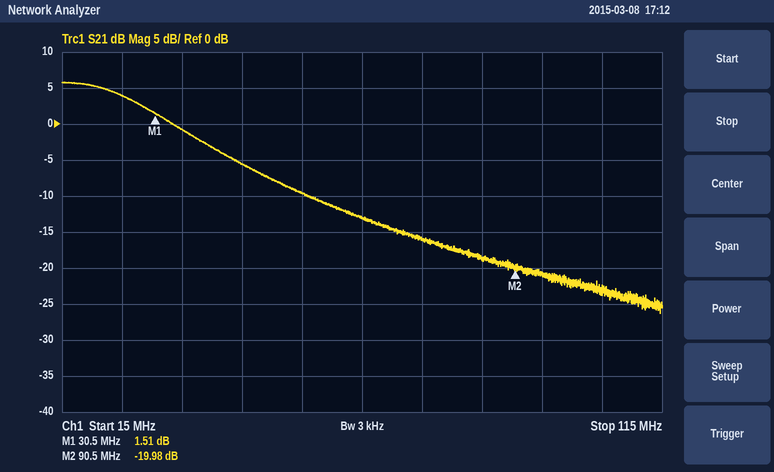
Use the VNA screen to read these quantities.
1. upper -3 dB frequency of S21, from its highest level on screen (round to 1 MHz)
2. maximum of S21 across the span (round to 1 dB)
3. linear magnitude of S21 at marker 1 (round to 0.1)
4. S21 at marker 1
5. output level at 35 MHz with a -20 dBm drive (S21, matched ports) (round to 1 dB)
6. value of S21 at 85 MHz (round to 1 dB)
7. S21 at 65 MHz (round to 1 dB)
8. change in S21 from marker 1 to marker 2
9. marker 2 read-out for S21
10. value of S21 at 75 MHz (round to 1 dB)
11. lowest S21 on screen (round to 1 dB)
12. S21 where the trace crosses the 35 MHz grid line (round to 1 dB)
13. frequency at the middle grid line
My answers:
28 MHz
6 dB
1.2
1.51 dB
-21 dBm
-19 dB
-13 dB
-21.49 dB
-19.98 dB
-16 dB
-26 dB
-1 dB
65 MHz
